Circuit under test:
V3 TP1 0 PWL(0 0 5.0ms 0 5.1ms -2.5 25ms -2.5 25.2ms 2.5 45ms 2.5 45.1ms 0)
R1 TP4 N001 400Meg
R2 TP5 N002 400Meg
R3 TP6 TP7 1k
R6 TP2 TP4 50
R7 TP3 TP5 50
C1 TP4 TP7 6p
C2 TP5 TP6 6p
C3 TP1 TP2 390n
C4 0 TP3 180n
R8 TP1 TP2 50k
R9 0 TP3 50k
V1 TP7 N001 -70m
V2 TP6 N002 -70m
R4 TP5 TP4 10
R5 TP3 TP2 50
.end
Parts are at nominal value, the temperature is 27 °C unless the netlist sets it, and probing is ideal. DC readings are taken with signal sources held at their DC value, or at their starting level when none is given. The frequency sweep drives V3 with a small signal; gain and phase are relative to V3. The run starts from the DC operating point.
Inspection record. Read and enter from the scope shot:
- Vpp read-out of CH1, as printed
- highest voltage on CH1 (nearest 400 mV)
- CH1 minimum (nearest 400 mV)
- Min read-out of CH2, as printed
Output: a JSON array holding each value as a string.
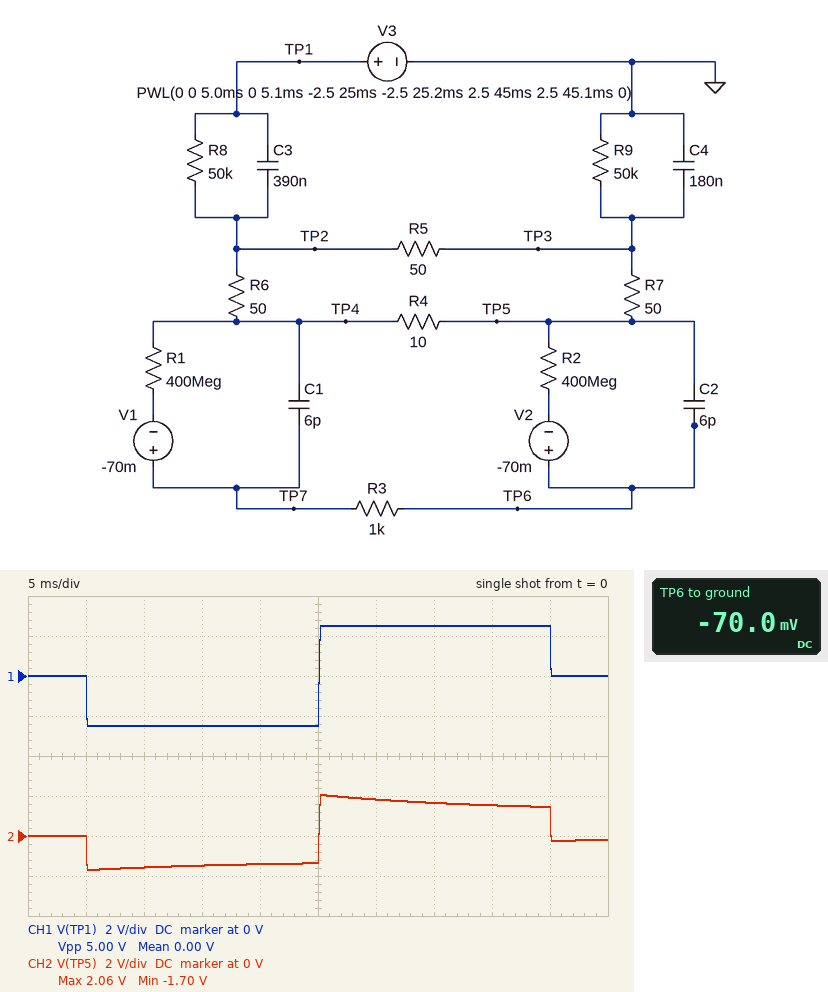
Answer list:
["5.00 V", "2.4 V", "-2.4 V", "-1.70 V"]
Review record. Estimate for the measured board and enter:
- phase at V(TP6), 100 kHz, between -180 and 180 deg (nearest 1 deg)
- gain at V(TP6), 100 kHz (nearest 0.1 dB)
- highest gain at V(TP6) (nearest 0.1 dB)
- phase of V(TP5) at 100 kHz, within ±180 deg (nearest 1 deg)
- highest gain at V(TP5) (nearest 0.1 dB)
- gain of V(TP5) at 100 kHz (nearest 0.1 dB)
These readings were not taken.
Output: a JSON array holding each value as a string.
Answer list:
["-7 deg", "-5.6 dB", "-3.3 dB", "-9 deg", "-3.3 dB", "-6.2 dB"]
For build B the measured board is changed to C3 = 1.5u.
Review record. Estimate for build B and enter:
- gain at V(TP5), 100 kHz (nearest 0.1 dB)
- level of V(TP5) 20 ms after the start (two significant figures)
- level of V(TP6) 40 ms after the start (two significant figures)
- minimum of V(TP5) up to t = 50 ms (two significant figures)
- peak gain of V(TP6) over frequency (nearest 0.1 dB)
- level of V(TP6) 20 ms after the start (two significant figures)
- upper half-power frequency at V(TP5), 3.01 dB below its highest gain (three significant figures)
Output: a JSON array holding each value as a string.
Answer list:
["-6.0 dB", "-1.9 V", "2.1 V", "-2.2 V", "-1.0 dB", "-2.0 V", "41.6 kHz"]
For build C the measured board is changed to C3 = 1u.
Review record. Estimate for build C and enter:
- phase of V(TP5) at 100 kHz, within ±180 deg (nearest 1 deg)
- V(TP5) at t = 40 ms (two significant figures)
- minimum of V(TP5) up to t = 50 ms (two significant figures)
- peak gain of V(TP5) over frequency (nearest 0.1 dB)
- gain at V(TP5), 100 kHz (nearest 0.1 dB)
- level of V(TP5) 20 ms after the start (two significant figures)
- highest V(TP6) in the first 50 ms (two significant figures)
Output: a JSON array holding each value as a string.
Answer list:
["-13 deg", "2.0 V", "-2.1 V", "-1.4 dB", "-6.0 dB", "-1.8 V", "2.5 V"]
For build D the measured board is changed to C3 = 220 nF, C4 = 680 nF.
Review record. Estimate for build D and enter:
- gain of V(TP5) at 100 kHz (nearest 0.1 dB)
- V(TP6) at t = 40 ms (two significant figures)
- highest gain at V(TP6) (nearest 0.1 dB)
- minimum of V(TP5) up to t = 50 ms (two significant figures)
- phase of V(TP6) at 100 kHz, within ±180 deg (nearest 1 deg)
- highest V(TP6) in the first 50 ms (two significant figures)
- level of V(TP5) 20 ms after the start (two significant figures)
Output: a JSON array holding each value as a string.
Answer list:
["-7.1 dB", "660 mV", "-6.0 dB", "-990 mV", "8 deg", "760 mV", "-920 mV"]
